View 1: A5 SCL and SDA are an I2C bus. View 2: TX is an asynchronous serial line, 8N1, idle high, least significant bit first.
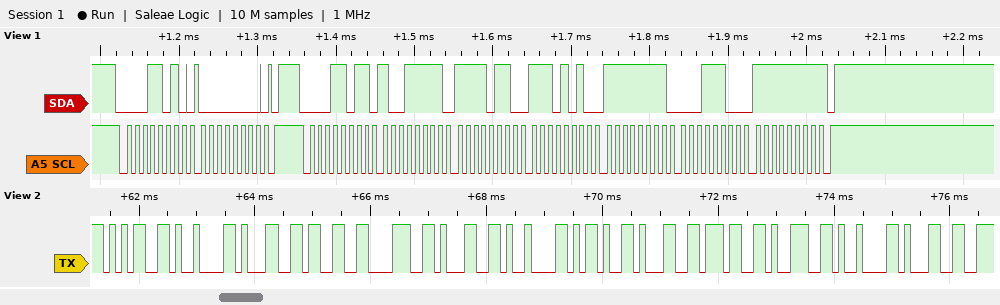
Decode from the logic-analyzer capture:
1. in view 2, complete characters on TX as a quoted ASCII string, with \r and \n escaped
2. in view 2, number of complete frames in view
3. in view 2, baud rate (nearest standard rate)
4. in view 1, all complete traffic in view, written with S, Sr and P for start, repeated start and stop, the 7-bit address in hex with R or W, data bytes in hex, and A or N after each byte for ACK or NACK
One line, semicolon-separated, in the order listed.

"5\t1381\t-179\t1"; 13; 9600 baud; S 0DW A 00 A P S 0DR A 9F A F6 A EA A FF A 1C A FF N P
